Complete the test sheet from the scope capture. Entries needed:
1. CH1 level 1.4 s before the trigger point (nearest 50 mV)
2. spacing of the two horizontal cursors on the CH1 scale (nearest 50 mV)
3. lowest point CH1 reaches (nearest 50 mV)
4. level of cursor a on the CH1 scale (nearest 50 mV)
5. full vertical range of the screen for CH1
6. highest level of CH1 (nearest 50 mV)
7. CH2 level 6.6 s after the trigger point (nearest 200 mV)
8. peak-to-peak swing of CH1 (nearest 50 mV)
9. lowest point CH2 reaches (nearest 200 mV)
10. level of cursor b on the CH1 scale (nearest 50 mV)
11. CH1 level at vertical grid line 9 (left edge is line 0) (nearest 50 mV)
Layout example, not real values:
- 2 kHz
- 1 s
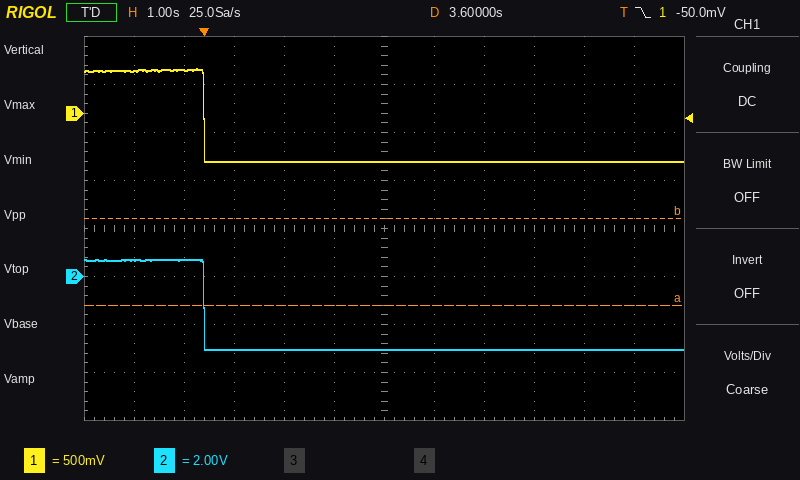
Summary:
- 450 mV
- 900 mV
- -500 mV
- -2.00 V
- 4 V
- 450 mV
- -3.0 V
- 950 mV
- -3.0 V
- -1.10 V
- -500 mV
